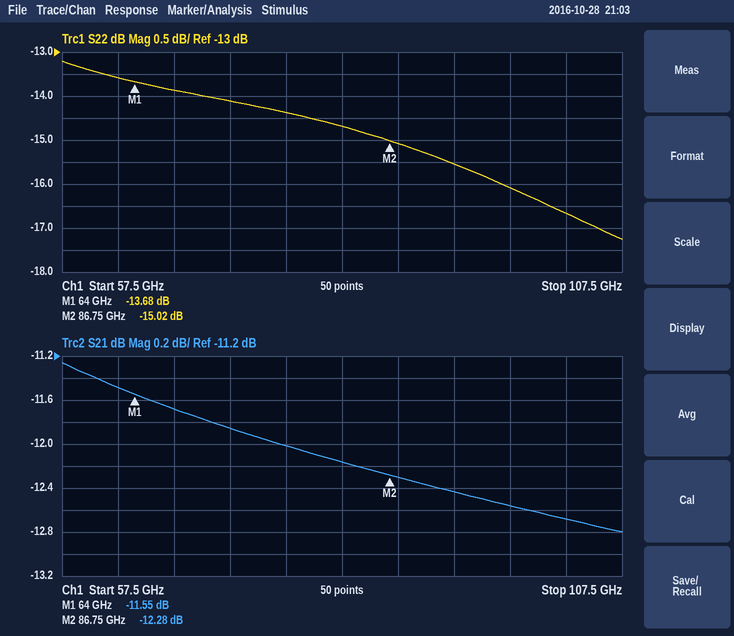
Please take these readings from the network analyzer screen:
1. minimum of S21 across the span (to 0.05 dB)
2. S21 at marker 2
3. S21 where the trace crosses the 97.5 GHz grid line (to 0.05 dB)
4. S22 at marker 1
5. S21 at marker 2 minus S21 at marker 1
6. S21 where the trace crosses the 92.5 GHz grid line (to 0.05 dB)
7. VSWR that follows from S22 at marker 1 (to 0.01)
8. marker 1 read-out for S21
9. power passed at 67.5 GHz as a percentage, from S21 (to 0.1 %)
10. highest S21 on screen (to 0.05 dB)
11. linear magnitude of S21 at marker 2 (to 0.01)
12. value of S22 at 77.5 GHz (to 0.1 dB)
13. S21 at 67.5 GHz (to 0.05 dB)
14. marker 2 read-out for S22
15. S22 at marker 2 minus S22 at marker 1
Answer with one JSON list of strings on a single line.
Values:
["-12.80 dB", "-12.28 dB", "-12.55 dB", "-13.68 dB", "-0.73 dB", "-12.45 dB", "1.52", "-11.55 dB", "6.8 %", "-11.25 dB", "0.24", "-14.4 dB", "-11.70 dB", "-15.02 dB", "-1.34 dB"]
